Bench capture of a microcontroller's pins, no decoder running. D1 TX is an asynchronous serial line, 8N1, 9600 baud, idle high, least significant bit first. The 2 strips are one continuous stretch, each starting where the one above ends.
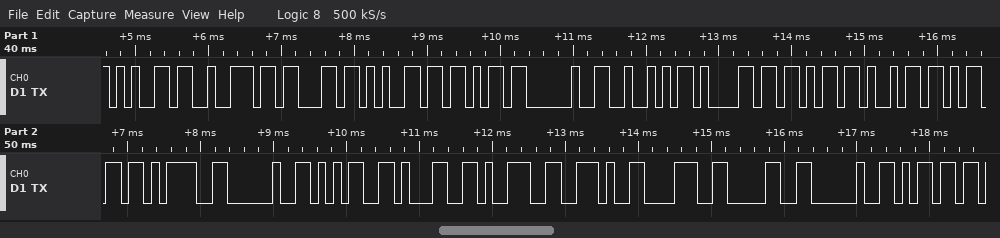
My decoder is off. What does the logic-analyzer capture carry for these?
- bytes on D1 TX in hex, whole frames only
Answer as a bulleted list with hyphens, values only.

- 65 72 63 65 6B 20 52 61 6B 69 6D 3D 20 35 31 39 2E 38 30 20 6D
